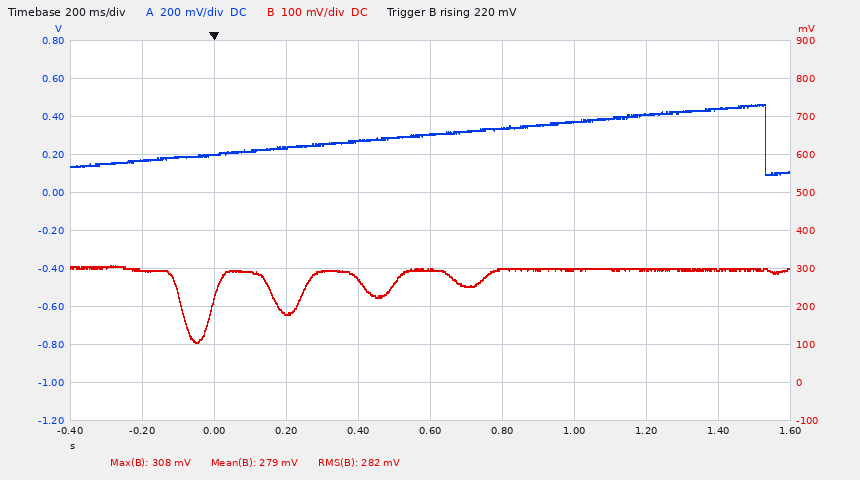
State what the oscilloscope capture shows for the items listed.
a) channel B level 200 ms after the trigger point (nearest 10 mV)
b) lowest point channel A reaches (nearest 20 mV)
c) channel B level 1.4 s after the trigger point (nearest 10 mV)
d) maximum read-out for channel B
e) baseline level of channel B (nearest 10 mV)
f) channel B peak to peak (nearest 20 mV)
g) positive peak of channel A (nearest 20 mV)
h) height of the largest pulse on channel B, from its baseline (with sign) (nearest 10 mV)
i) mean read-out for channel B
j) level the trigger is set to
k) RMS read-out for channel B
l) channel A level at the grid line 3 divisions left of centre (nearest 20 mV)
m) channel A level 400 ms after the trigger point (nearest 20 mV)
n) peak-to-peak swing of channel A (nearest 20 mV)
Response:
180 mV
100 mV
300 mV
308 mV
300 mV
200 mV
460 mV
-190 mV
279 mV
220 mV
282 mV
200 mV
280 mV
360 mV
